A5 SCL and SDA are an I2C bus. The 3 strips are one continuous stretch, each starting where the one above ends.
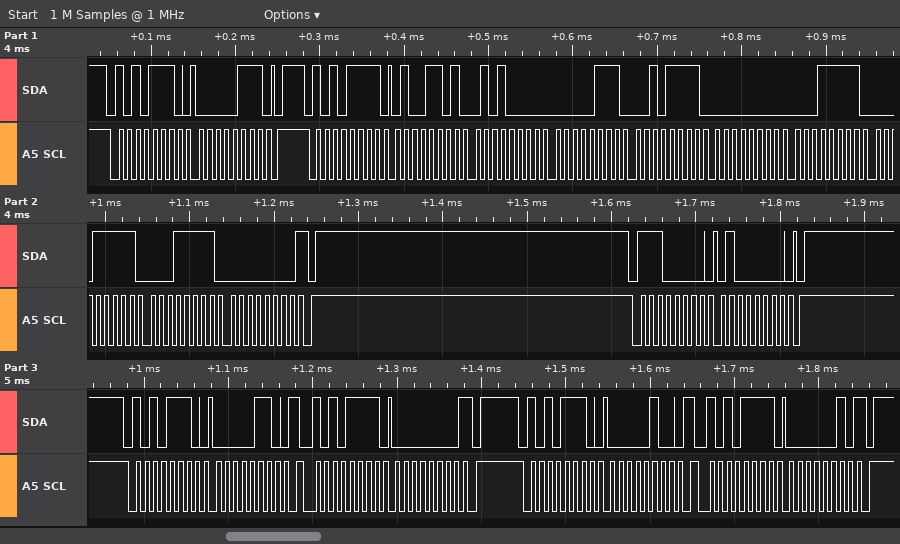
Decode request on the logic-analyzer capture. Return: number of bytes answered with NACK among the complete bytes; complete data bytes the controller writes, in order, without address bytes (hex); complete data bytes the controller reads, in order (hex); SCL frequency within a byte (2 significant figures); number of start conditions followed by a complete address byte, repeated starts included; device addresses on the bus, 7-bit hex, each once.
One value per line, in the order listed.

3
07 40 06 04
4D 50 07 2F 00 1F 1F 1F 00 00 02
100 kHz
7
0x57 0x70
